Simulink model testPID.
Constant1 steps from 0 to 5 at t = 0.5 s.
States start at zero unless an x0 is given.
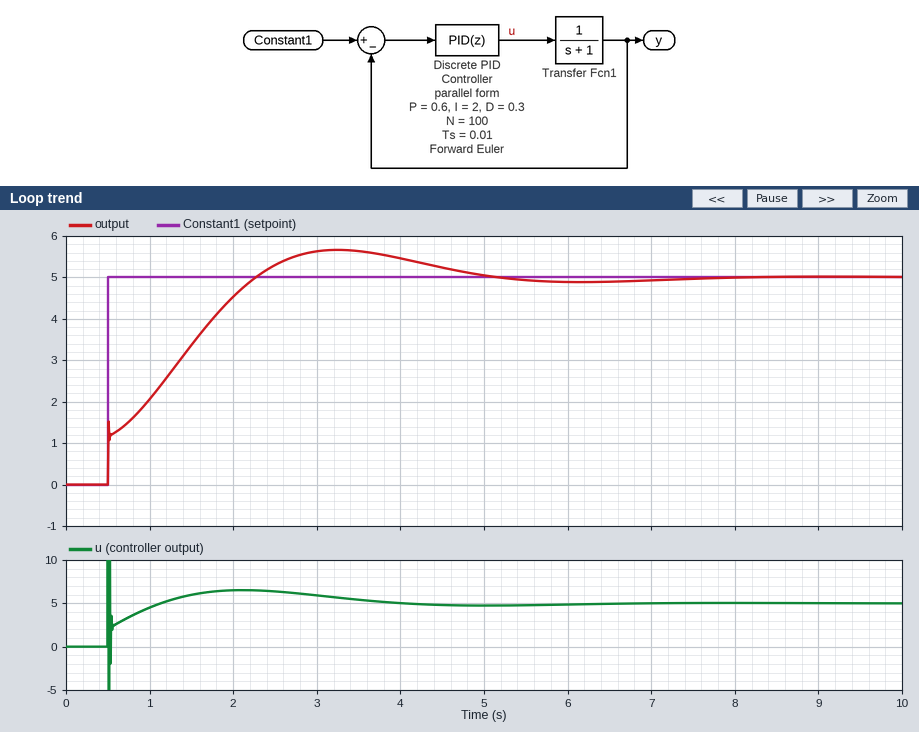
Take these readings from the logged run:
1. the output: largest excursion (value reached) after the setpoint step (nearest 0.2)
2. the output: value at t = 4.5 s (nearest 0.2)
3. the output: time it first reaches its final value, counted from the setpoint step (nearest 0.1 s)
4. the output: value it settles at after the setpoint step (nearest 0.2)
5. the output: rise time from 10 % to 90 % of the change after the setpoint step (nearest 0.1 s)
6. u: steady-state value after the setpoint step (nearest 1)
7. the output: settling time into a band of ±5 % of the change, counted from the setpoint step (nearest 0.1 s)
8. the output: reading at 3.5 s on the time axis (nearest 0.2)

5.6
5.2
1.8 s
5.0
1.5 s
5
4.0 s
5.6
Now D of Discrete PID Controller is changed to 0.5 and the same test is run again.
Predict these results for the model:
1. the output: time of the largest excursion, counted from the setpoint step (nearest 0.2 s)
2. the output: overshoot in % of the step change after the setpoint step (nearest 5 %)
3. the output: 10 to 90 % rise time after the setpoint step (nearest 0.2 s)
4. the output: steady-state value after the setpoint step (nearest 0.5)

3.0 s
15 %
1.6 s
5.0
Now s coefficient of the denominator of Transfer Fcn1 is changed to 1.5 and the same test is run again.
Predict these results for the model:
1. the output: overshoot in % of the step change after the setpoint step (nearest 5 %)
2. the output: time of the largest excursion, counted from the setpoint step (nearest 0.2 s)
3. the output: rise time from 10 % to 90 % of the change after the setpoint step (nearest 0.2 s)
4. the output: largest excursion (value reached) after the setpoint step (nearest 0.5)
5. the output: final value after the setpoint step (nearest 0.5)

20 %
3.0 s
1.6 s
6.0
5.0
